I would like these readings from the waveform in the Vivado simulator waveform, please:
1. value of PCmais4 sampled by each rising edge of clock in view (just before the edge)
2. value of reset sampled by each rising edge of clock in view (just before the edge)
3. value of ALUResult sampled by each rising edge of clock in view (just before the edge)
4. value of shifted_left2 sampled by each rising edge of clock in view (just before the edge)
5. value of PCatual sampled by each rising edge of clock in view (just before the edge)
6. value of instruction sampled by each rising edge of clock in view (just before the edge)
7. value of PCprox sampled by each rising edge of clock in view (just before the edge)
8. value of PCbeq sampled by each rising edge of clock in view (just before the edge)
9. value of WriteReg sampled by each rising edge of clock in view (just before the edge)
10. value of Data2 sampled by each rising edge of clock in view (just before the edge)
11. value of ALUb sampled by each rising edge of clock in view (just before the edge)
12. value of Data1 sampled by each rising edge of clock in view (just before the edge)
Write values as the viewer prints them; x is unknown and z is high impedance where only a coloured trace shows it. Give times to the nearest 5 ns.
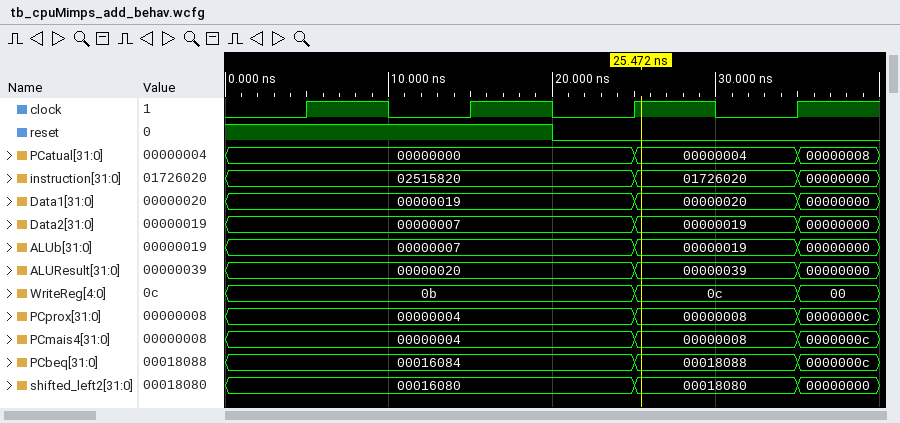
00000004, 00000004, 00000004, 00000008
1 1 0 0
00000020, 00000020, 00000020, 00000039
00016080, 00016080, 00016080, 00018080
00000000, 00000000, 00000000, 00000004
02515820, 02515820, 02515820, 01726020
00000004, 00000004, 00000004, 00000008
00016084, 00016084, 00016084, 00018088
0b, 0b, 0b, 0c
00000007, 00000007, 00000007, 00000019
00000007, 00000007, 00000007, 00000019
00000019, 00000019, 00000019, 00000020
